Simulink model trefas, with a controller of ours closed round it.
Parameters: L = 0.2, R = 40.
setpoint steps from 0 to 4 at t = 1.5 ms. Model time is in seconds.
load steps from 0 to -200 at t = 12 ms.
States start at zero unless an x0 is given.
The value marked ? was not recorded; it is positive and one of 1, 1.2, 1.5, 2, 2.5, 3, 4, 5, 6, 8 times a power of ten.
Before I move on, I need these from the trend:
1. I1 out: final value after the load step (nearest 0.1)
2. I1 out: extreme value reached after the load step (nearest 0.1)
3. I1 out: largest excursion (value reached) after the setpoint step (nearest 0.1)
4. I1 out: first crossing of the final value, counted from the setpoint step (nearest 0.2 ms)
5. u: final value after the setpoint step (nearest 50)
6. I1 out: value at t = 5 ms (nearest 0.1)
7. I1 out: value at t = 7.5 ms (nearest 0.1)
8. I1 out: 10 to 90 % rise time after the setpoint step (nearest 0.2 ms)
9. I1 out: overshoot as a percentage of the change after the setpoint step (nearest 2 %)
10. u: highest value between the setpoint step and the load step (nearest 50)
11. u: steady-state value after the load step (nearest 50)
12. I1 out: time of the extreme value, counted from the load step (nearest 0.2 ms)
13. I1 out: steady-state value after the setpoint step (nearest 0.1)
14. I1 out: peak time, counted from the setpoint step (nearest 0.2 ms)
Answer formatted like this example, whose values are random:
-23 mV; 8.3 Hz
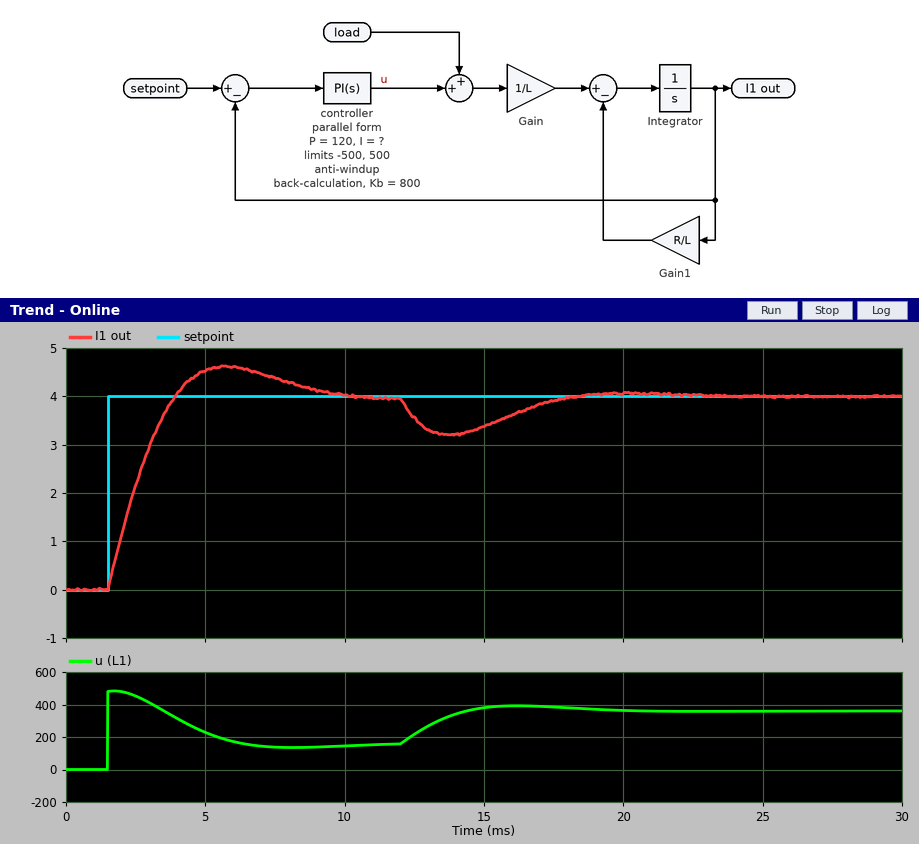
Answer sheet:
4.0; 3.2; 4.6; 2.4 ms; 150; 4.5; 4.4; 1.8 ms; 16 %; 500; 350; 1.8 ms; 4.0; 4.2 ms
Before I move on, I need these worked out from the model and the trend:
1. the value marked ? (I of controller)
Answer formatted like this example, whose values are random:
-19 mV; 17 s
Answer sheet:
80000
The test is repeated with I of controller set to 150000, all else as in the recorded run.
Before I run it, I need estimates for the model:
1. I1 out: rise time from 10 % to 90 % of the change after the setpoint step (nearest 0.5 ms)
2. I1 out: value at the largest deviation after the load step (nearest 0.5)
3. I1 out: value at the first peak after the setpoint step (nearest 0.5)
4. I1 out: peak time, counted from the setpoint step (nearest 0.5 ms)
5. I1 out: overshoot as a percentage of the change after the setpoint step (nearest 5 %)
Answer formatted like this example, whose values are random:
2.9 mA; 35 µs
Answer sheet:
1.5 ms; 3.5; 5.0; 3.5 ms; 25 %
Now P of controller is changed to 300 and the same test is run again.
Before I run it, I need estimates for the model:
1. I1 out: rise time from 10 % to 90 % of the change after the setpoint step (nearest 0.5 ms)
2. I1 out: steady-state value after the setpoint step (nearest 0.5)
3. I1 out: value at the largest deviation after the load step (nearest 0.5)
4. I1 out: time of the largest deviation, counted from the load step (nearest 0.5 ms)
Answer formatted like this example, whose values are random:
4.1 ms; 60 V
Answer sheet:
2.5 ms; 4.0; 3.5; 1.5 ms
